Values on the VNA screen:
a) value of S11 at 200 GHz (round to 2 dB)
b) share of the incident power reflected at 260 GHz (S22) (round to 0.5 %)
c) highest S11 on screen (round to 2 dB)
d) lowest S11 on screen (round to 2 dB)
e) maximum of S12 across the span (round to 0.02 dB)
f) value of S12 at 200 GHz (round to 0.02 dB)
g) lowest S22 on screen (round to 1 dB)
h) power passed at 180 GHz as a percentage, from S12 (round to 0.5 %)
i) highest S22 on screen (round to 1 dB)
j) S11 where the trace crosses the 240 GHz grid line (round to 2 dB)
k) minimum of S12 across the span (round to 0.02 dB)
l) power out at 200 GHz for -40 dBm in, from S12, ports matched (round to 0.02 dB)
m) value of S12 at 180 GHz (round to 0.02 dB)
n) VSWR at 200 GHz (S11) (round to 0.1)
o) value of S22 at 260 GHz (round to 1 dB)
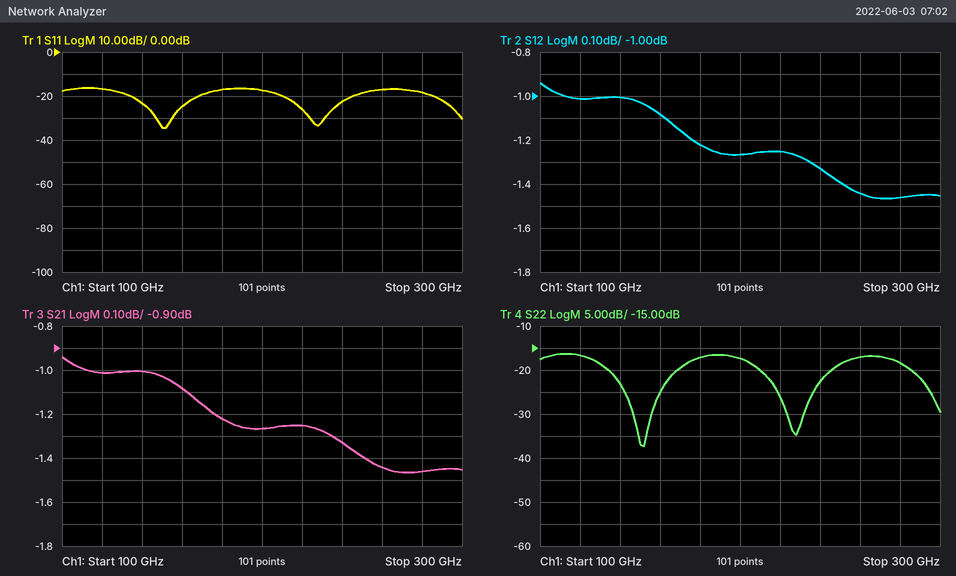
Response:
-18 dB
2.0 %
-16 dB
-34 dB
-0.94 dB
-1.26 dB
-37 dB
75.5 %
-16 dB
-22 dB
-1.46 dB
-41.26 dBm
-1.22 dB
1.3
-17 dB
